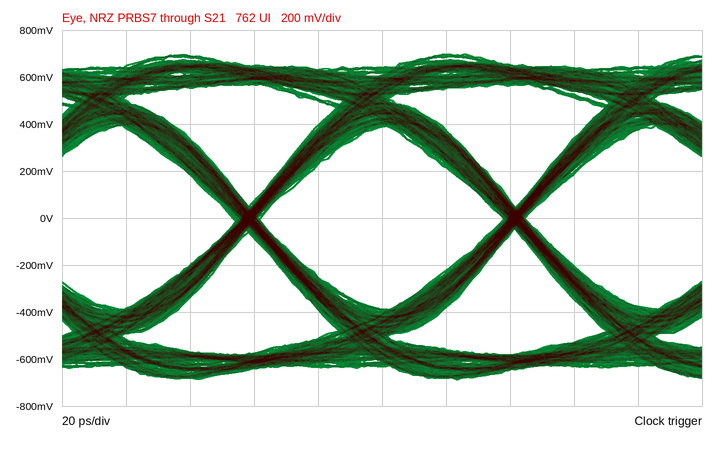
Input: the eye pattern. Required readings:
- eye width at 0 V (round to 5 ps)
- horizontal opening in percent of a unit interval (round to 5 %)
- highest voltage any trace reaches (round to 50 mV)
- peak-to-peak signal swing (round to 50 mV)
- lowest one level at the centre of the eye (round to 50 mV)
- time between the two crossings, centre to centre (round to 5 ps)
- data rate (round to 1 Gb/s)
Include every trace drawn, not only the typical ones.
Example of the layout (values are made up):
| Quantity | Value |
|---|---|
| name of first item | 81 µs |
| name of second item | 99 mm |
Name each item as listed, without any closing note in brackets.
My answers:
| Quantity | Value |
|---|---|
| eye width at 0 V | 75 ps |
| horizontal opening in percent of a unit interval | 90 % |
| highest voltage any trace reaches | 700 mV |
| peak-to-peak signal swing | 1.40 V |
| lowest one level at the centre of the eye | 400 mV |
| time between the two crossings, centre to centre | 85 ps |
| data rate | 12 Gb/s |
